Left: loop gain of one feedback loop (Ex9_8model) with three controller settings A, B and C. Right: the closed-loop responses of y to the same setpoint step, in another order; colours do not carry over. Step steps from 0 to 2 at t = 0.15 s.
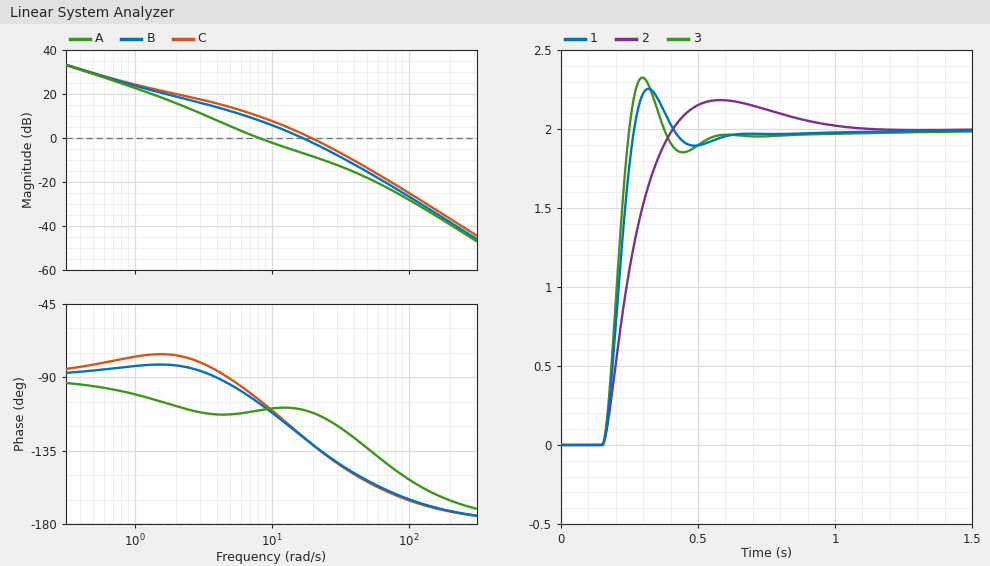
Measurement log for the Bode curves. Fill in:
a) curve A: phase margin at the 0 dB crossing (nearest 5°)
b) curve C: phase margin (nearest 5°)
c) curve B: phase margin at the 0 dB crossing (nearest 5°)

70°
50°
55°
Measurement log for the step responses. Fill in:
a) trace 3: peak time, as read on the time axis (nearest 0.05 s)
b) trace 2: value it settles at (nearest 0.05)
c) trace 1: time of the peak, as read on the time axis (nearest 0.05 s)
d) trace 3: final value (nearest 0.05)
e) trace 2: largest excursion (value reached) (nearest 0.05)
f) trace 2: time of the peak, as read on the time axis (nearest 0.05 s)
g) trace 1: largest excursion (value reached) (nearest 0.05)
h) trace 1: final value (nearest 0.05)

0.30 s
2.00
0.30 s
2.00
2.20
0.60 s
2.25
2.00
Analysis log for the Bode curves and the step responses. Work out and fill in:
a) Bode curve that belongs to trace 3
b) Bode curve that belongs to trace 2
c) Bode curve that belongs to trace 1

C
A
B
